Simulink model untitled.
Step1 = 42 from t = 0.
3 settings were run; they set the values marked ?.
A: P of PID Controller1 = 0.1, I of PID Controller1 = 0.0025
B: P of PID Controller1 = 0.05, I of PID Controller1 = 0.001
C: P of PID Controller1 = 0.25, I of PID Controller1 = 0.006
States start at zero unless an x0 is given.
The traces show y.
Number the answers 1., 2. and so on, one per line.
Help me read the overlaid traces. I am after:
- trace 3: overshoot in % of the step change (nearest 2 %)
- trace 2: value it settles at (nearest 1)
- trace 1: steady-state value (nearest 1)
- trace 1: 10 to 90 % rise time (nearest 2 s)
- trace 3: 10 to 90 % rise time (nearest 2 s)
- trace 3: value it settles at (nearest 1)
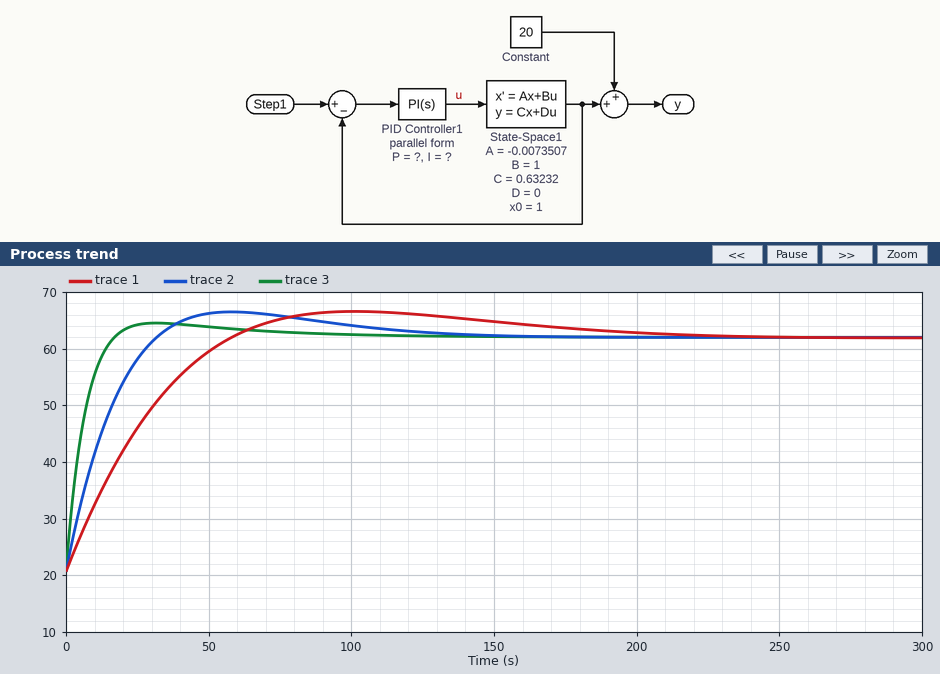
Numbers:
1. 6 %
2. 62
3. 62
4. 42 s
5. 12 s
6. 62
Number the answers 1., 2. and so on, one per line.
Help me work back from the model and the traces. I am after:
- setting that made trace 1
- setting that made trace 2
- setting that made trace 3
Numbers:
1. B
2. A
3. C
